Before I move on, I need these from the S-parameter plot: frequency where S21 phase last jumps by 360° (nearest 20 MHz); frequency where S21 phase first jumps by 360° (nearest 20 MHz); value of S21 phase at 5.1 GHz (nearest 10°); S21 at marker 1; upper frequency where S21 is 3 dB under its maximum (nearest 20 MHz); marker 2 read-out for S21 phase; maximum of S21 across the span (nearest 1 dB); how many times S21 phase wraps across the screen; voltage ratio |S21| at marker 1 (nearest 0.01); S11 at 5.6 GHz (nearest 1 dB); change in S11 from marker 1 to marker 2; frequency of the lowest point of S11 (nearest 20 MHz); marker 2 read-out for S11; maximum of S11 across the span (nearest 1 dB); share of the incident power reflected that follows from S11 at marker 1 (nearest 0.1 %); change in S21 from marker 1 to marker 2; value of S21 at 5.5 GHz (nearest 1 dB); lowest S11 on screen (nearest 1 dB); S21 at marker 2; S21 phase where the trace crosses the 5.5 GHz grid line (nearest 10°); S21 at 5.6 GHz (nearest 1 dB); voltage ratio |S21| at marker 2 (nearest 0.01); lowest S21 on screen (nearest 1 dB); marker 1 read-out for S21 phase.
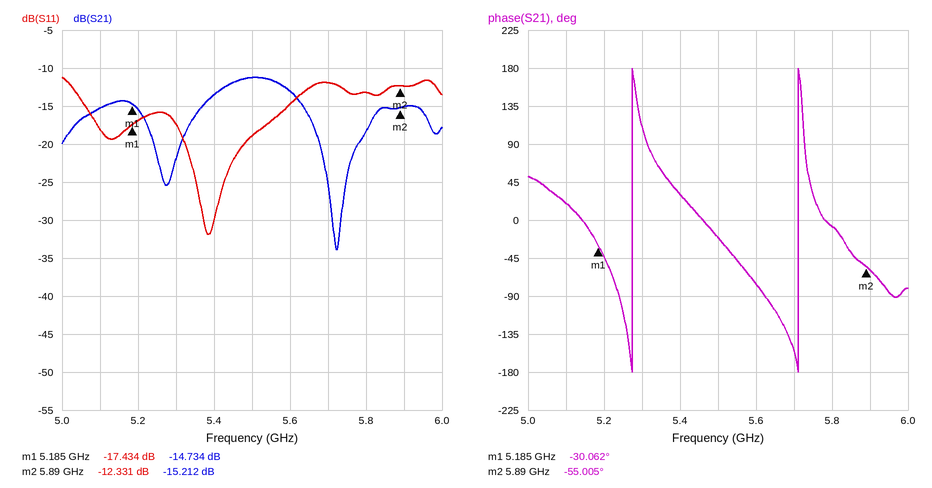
5.72 GHz
5.28 GHz
20°
-14.734 dB
5.62 GHz
-55.005°
-11 dB
2
0.18
-15 dB
5.103 dB
5.38 GHz
-12.331 dB
-11 dB
1.8 %
-0.478 dB
-11 dB
-32 dB
-15.212 dB
-20°
-13 dB
0.17
-34 dB
-30.062°
